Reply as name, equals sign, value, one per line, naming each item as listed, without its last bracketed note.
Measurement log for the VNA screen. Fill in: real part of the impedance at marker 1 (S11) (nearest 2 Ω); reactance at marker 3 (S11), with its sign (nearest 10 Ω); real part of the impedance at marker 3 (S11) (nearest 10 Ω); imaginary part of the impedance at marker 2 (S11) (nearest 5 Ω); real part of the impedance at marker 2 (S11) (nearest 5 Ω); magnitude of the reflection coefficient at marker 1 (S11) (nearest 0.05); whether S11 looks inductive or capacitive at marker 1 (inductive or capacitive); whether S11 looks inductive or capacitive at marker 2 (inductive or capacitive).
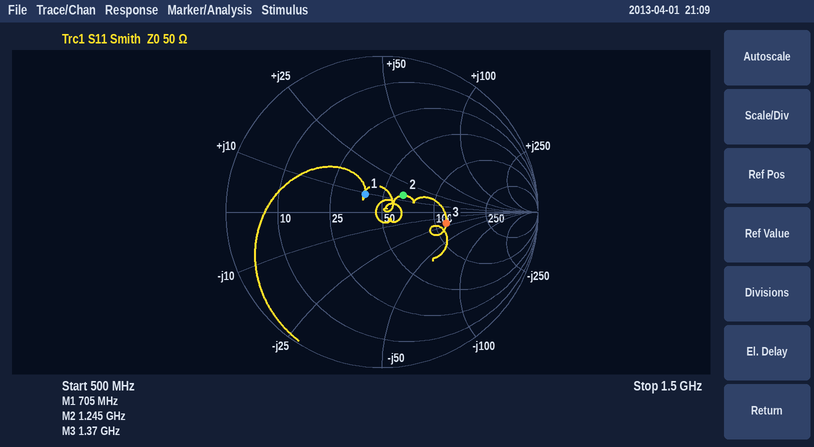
real part of the impedance at marker 1 (S11) = 40 Ω
reactance at marker 3 (S11), with its sign = -20 Ω
real part of the impedance at marker 3 (S11) = 120 Ω
imaginary part of the impedance at marker 2 (S11) = +15 Ω
real part of the impedance at marker 2 (S11) = 65 Ω
magnitude of the reflection coefficient at marker 1 (S11) = 0.15
whether S11 looks inductive or capacitive at marker 1 = inductive
whether S11 looks inductive or capacitive at marker 2 = inductive
